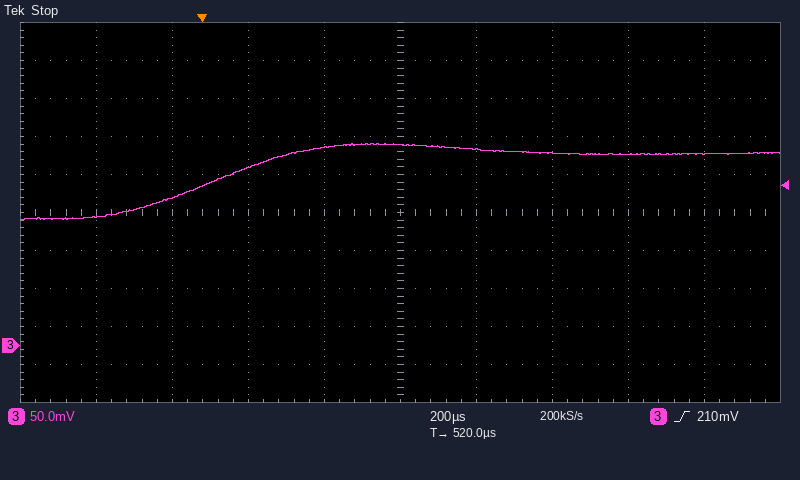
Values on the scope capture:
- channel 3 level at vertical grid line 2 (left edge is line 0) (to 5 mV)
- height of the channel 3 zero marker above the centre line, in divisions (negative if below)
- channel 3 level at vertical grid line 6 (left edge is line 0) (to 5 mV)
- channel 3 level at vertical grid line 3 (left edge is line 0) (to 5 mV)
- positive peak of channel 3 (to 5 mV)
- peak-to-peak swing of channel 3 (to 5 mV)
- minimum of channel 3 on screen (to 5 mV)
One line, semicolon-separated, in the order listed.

195 mV; -3.5 div; 260 mV; 235 mV; 265 mV; 100 mV; 165 mV
